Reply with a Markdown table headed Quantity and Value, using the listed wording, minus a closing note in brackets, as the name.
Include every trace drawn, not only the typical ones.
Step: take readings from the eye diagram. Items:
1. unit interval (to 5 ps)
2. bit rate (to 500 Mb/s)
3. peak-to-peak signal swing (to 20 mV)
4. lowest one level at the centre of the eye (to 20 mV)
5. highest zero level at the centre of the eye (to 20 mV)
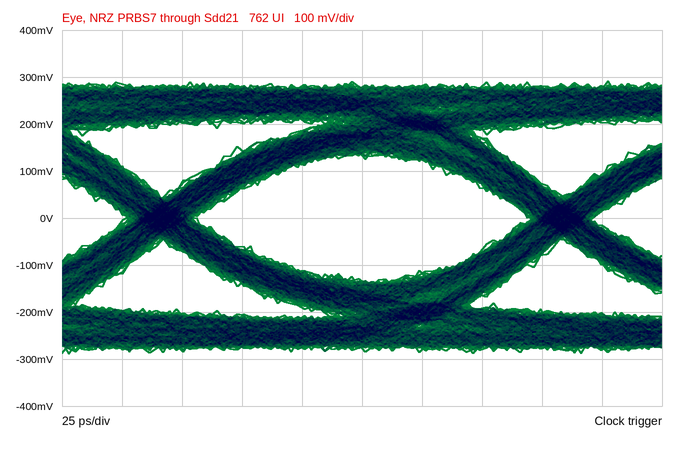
| Quantity | Value |
|---|---|
| unit interval | 165 ps |
| bit rate | 6.0 Gb/s |
| peak-to-peak signal swing | 580 mV |
| lowest one level at the centre of the eye | 140 mV |
| highest zero level at the centre of the eye | -140 mV |
